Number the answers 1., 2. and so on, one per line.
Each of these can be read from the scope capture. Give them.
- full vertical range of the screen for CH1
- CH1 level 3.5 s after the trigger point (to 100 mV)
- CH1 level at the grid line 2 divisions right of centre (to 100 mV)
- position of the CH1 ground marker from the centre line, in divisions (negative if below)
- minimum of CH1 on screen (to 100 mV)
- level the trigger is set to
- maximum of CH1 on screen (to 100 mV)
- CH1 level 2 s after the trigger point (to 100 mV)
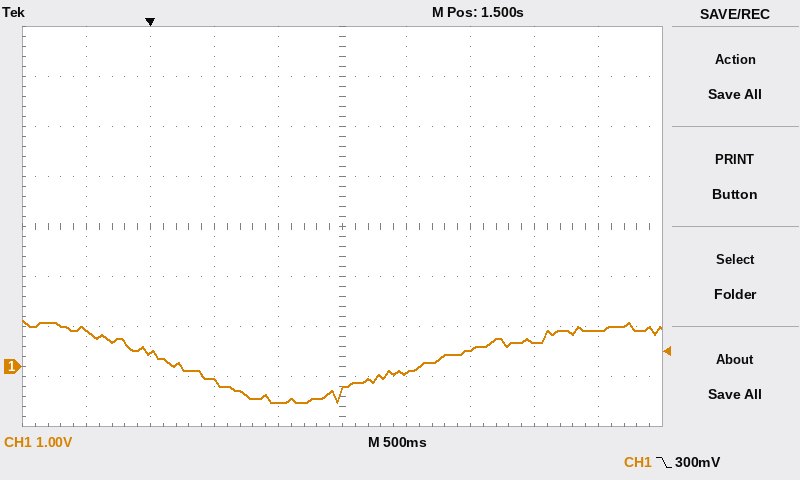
1. 8 V
2. 700 mV
3. 300 mV
4. -2.8 div
5. -700 mV
6. 300 mV
7. 900 mV
8. -100 mV
